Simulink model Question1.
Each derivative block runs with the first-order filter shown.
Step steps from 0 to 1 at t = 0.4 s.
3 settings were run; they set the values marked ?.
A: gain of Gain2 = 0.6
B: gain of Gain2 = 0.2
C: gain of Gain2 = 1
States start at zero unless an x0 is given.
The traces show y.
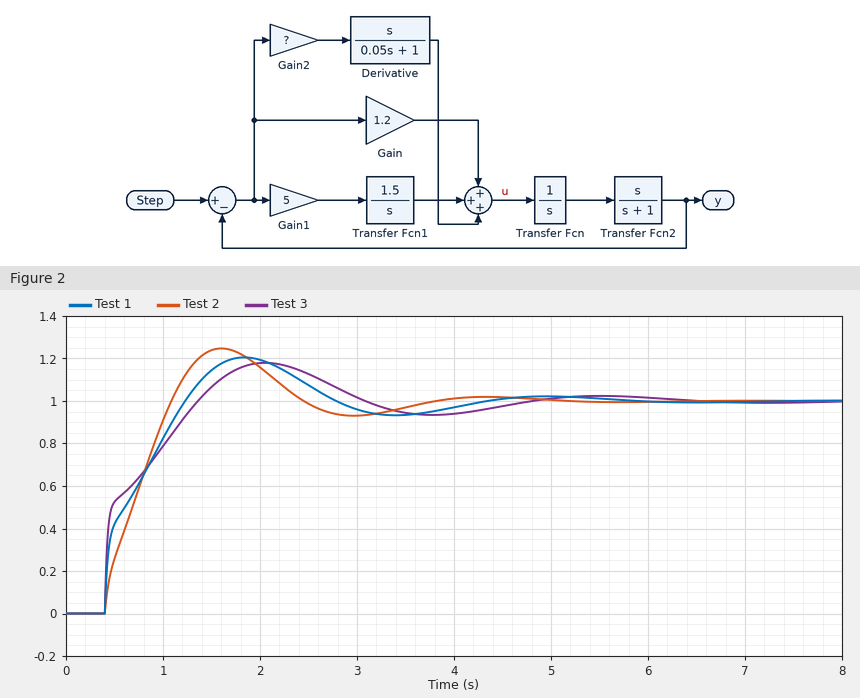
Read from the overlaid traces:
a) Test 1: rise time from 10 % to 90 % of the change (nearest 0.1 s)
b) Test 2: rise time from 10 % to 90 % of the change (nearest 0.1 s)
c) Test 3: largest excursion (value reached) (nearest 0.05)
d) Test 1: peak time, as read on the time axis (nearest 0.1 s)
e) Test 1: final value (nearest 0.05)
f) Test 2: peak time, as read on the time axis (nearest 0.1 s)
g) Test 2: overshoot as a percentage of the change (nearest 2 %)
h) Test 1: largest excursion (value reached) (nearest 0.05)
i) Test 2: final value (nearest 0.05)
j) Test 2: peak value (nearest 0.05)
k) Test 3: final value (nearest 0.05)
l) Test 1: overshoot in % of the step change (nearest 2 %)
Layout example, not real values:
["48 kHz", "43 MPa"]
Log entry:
["0.7 s", "0.6 s", "1.20", "1.8 s", "1.00", "1.6 s", "24 %", "1.20", "1.00", "1.25", "1.00", "20 %"]
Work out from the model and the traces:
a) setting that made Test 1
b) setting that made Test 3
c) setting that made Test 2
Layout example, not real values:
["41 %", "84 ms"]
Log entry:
["A", "C", "B"]
